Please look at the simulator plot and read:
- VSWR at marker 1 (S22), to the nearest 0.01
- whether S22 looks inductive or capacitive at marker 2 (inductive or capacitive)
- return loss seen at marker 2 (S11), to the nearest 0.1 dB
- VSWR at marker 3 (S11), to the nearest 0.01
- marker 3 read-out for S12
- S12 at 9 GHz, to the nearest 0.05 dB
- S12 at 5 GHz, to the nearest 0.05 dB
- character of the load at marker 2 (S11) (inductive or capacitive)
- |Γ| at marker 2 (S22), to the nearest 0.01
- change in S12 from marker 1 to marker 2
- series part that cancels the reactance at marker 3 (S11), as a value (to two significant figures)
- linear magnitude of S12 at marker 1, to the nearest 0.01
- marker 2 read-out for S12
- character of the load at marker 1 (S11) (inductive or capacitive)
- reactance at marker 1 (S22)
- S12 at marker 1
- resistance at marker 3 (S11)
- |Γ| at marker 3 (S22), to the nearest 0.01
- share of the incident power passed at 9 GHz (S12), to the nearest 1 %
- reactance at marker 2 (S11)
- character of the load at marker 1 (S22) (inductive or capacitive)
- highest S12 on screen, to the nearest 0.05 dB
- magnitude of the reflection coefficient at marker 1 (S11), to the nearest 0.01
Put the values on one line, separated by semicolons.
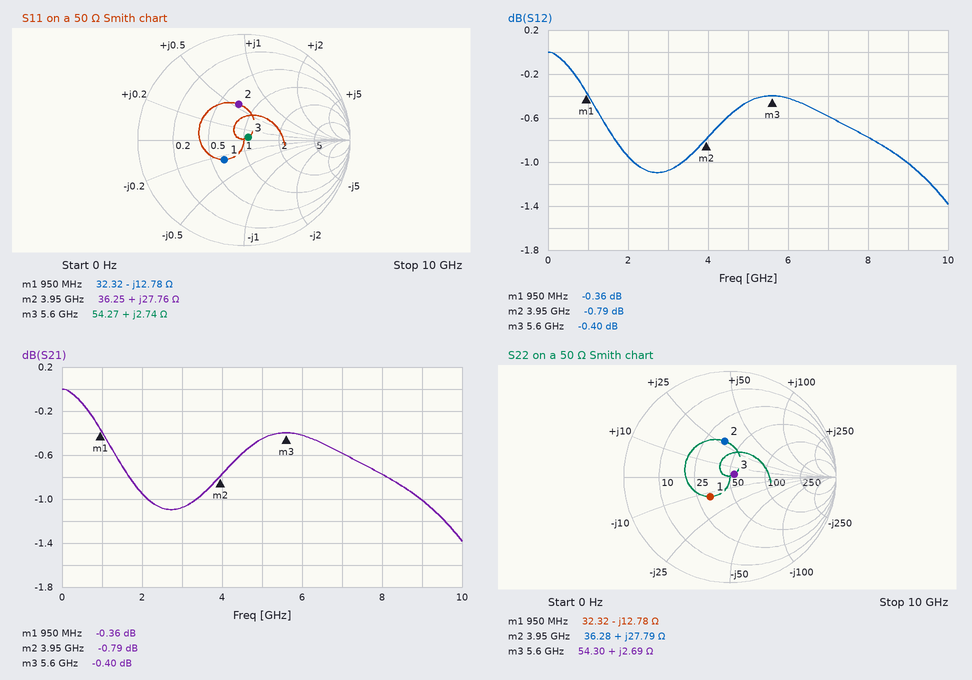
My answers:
1.71; inductive; 9.3 dB; 1.10; -0.40 dB; -1.00 dB; -0.45 dB; inductive; 0.34; -0.43 dB; 10 pF; 0.96; -0.79 dB; capacitive; -12.78 Ω; -0.36 dB; 54.27 Ω; 0.05; 79 %; +27.76 Ω; capacitive; 0.00 dB; 0.26
